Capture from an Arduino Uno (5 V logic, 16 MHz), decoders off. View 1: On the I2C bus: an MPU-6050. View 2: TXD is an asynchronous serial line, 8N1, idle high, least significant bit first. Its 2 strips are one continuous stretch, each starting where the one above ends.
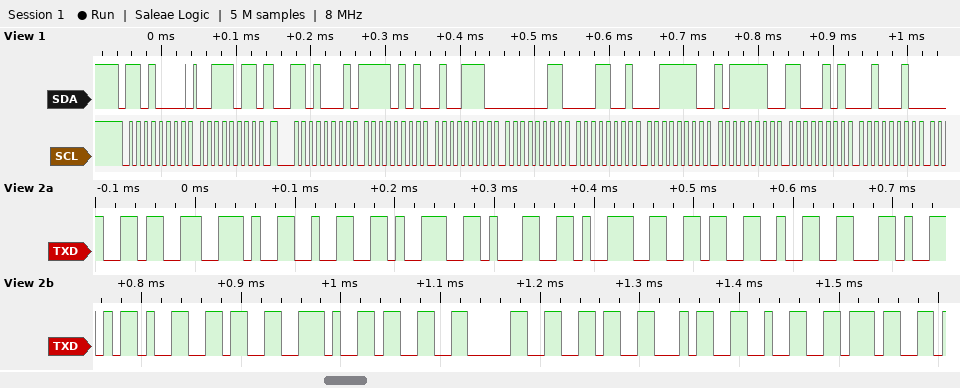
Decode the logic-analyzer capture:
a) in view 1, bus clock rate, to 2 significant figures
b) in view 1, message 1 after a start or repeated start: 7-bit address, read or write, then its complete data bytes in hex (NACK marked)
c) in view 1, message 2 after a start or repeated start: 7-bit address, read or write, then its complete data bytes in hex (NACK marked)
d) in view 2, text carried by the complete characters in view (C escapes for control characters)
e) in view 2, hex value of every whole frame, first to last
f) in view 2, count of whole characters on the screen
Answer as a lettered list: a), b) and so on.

a) 100 kHz
b) 0x68 write: 3B
c) 0x68 read: F5 4E 03 19 3E BE C5 22
d) "6.291962,-6.306427"
e) 36 2E 32 39 31 39 36 32 2C 2D 36 2E 33 30 36 34 32 37
f) 18
